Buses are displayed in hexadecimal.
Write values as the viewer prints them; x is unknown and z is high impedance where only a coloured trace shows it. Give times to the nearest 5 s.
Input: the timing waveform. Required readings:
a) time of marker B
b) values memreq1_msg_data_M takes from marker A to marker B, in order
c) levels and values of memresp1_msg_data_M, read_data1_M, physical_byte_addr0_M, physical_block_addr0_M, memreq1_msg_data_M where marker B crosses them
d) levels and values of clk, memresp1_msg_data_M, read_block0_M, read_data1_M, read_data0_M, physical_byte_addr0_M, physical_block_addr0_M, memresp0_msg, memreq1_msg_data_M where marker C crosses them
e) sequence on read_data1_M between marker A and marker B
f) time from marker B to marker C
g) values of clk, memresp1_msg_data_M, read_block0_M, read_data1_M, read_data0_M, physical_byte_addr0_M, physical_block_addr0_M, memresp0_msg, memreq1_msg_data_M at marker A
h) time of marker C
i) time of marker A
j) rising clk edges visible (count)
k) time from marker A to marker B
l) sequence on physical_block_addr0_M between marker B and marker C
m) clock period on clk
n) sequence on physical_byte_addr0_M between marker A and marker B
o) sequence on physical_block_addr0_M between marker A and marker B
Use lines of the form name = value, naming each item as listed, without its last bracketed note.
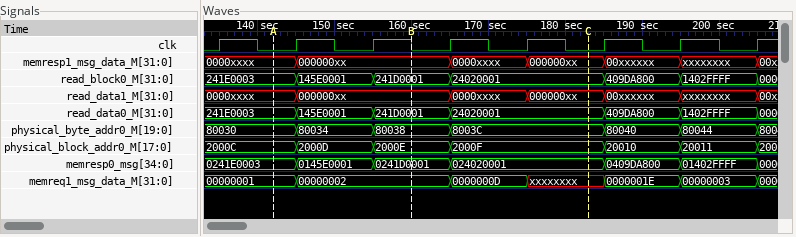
time of marker B = 160 s
values memreq1_msg_data_M takes from marker A to marker B, in order = 00000001, 00000002
levels and values of memresp1_msg_data_M, read_data1_M, physical_byte_addr0_M, physical_block_addr0_M, memreq1_msg_data_M where marker B crosses them = memresp1_msg_data_M=000000xx, read_data1_M=000000xx, physical_byte_addr0_M=80038, physical_block_addr0_M=2000E, memreq1_msg_data_M=00000002
levels and values of clk, memresp1_msg_data_M, read_block0_M, read_data1_M, read_data0_M, physical_byte_addr0_M, physical_block_addr0_M, memresp0_msg, memreq1_msg_data_M where marker C crosses them = clk=0, memresp1_msg_data_M=000000xx, read_block0_M=24020001, read_data1_M=000000xx, read_data0_M=24020001, physical_byte_addr0_M=8003C, physical_block_addr0_M=2000F, memresp0_msg=024020001, memreq1_msg_data_M=xxxxxxxx
sequence on read_data1_M between marker A and marker B = 0000xxxx, 000000xx
time from marker B to marker C = 25 s
values of clk, memresp1_msg_data_M, read_block0_M, read_data1_M, read_data0_M, physical_byte_addr0_M, physical_block_addr0_M, memresp0_msg, memreq1_msg_data_M at marker A = clk=0, memresp1_msg_data_M=0000xxxx, read_block0_M=241E0003, read_data1_M=0000xxxx, read_data0_M=241E0003, physical_byte_addr0_M=80030, physical_block_addr0_M=2000C, memresp0_msg=0241E0003, memreq1_msg_data_M=00000001
time of marker C = 185 s
time of marker A = 140 s
rising clk edges visible = 8
time from marker A to marker B = 20 s
sequence on physical_block_addr0_M between marker B and marker C = 2000E, 2000F
clock period on clk = 10 s
sequence on physical_byte_addr0_M between marker A and marker B = 80030, 80034, 80038
sequence on physical_block_addr0_M between marker A and marker B = 2000C, 2000D, 2000E
